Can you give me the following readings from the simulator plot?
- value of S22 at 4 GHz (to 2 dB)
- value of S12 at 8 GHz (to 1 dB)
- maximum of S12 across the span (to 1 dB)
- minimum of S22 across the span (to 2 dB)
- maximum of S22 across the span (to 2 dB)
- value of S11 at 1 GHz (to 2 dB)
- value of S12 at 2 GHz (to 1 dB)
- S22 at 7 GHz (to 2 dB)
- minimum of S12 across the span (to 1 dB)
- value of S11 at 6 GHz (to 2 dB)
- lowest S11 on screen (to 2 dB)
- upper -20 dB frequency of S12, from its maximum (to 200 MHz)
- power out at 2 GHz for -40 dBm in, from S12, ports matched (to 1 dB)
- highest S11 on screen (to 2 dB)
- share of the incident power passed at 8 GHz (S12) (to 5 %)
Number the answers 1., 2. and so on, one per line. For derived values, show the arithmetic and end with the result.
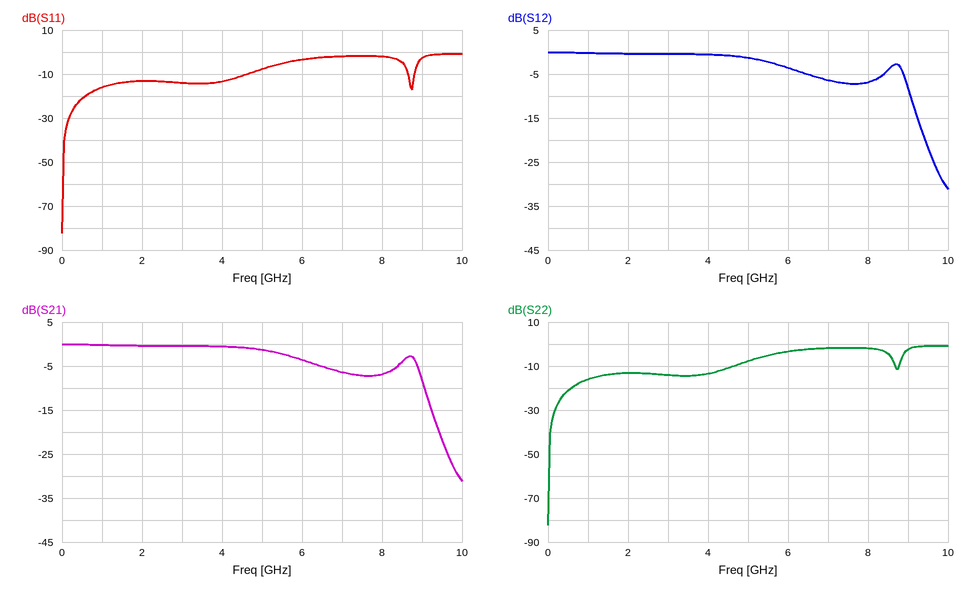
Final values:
1. -14 dB
2. -7 dB
3. 0 dB
4. -82 dB
5. 0 dB
6. -16 dB
7. 0 dB
8. -2 dB
9. -31 dB
10. -4 dB
11. -82 dB
12. 9.4 GHz
13. -40 dBm + (0 dB) = -40 dBm
14. 0 dB
15. 10^(-7/10) ≈ 20 %
